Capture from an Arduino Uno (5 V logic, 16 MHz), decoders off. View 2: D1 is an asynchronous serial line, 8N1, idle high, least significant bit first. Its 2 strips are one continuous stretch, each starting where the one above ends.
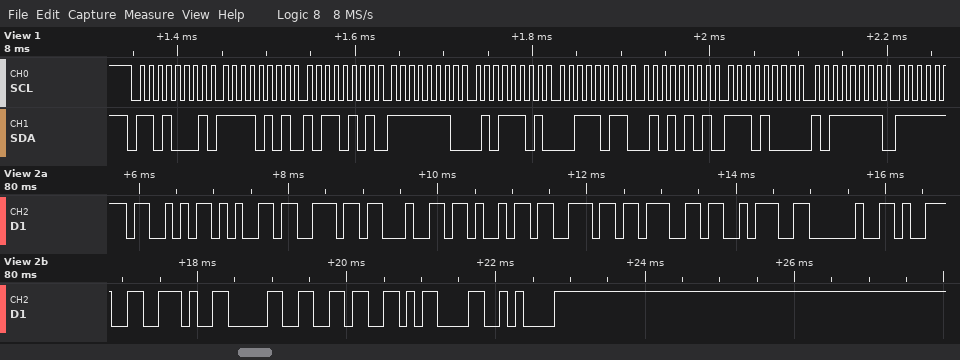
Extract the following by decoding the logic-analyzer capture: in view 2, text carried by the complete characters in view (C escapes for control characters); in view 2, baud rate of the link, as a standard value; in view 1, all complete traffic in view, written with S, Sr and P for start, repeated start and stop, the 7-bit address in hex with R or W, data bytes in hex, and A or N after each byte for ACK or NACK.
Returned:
"Sending: 9.06\r\n"
9600 baud
S 68R A F5 A B5 A FE A 5D A 3B A 55 A E8 A BF A
